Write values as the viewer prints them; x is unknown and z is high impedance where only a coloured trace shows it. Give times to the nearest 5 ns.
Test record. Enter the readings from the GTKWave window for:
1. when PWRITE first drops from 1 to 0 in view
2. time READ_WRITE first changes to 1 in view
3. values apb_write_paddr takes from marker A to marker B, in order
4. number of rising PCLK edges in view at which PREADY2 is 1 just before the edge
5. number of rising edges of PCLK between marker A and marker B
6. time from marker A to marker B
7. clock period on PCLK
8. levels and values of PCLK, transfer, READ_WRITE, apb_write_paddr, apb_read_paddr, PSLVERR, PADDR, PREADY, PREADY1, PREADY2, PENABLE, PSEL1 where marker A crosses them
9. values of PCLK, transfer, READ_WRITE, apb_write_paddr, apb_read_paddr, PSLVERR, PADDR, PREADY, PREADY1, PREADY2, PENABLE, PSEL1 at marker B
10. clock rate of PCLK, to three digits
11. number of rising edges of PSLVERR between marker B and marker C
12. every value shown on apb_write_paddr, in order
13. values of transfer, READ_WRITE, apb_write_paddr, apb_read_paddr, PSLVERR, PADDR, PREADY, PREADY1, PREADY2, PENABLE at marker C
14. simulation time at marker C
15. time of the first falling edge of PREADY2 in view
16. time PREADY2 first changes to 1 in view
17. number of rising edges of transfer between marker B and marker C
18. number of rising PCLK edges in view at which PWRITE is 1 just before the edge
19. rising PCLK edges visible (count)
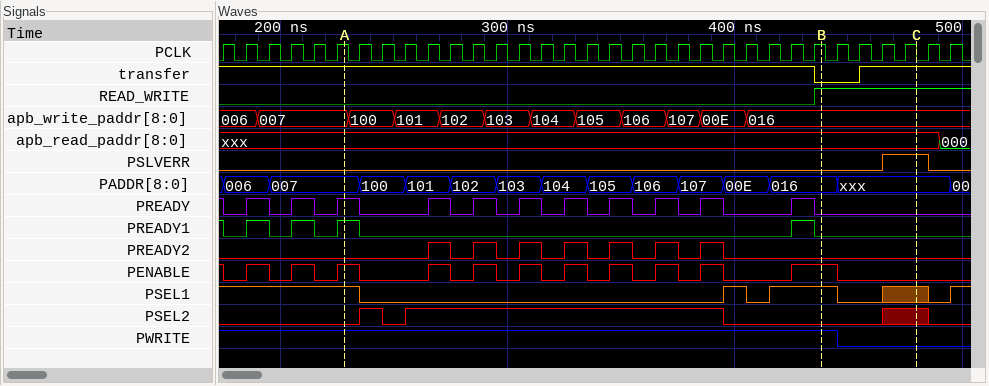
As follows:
445 ns
435 ns
007, 100, 101, 102, 103, 104, 105, 106, 107, 00E, 016
7
21
210 ns
10 ns
PCLK=1, transfer=1, READ_WRITE=0, apb_write_paddr=007, apb_read_paddr=xxx, PSLVERR=0, PADDR=007, PREADY=1, PREADY1=1, PREADY2=0, PENABLE=1, PSEL1=1
PCLK=1, transfer=0, READ_WRITE=1, apb_write_paddr=016, apb_read_paddr=xxx, PSLVERR=0, PADDR=016, PREADY=0, PREADY1=0, PREADY2=0, PENABLE=1, PSEL1=1
100 MHz
1
006, 007, 100, 101, 102, 103, 104, 105, 106, 107, 00E, 016
transfer=1, READ_WRITE=1, apb_write_paddr=016, apb_read_paddr=xxx, PSLVERR=1, PADDR=xxx, PREADY=0, PREADY1=0, PREADY2=0, PENABLE=0
480 ns
275 ns
265 ns
1
28
33
